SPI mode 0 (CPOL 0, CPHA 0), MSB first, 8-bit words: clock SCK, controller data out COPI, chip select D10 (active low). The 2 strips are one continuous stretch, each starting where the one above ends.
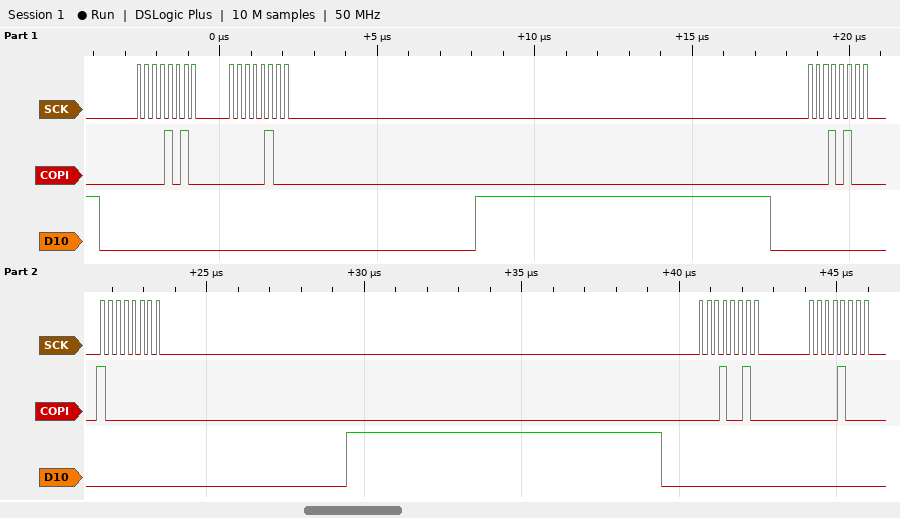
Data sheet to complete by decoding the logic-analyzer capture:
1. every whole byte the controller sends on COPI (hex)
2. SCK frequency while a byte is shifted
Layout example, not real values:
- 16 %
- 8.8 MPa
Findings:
- 0x0A 0x04 0x14 0x80 0x12 0x08
- 4 MHz
